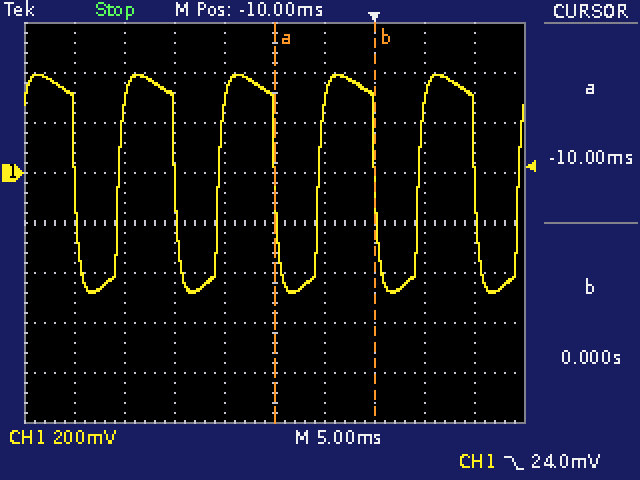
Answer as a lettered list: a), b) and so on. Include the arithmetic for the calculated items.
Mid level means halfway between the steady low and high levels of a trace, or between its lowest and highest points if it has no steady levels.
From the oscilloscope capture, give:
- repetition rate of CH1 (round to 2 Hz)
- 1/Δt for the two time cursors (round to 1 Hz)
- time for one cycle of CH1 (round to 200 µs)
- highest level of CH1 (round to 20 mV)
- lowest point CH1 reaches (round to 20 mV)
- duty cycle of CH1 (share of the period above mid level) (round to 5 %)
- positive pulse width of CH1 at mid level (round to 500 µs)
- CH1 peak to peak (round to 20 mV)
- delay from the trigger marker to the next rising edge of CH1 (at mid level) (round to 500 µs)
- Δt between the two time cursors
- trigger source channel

a) 1 / 10.0 ms ≈ 100 Hz
b) 1 / 10.0 ms ≈ 100 Hz
c) 10.0 ms
d) 400 mV
e) -480 mV
f) 5.5 ms / 10.0 ms ≈ 55 %
g) 5.5 ms
h) 400 mV − (-480 mV) = 880 mV
i) 4.5 ms
j) 0 s − (-10 ms) = 10.0 ms
k) CH1
